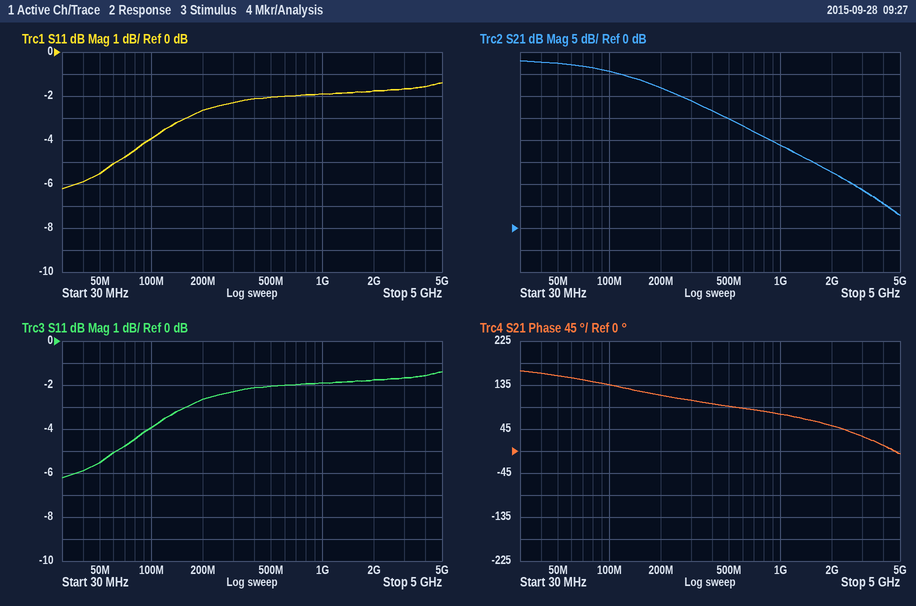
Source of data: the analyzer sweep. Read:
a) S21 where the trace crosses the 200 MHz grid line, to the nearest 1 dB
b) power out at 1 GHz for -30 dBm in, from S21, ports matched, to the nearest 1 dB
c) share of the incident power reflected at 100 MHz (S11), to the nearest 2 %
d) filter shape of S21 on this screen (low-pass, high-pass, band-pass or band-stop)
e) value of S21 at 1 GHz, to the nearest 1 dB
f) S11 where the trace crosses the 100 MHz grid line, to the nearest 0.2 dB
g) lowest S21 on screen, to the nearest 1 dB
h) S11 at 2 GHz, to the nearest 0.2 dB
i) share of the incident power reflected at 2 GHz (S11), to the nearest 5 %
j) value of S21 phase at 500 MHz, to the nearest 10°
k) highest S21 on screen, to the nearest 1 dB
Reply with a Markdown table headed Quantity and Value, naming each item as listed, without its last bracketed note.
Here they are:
| Quantity | Value |
|---|---|
| S21 where the trace crosses the 200 MHz grid line, to the nearest 1 dB | 32 dB |
| power out at 1 GHz for -30 dBm in, from S21, ports matched, to the nearest 1 dB | -11 dBm |
| share of the incident power reflected at 100 MHz (S11), to the nearest 2 % | 40 % |
| filter shape of S21 on this screen | low-pass |
| value of S21 at 1 GHz, to the nearest 1 dB | 19 dB |
| S11 where the trace crosses the 100 MHz grid line, to the nearest 0.2 dB | -4.0 dB |
| lowest S21 on screen, to the nearest 1 dB | 3 dB |
| S11 at 2 GHz, to the nearest 0.2 dB | -1.8 dB |
| share of the incident power reflected at 2 GHz (S11), to the nearest 5 % | 65 % |
| value of S21 phase at 500 MHz, to the nearest 10° | 90° |
| highest S21 on screen, to the nearest 1 dB | 38 dB |
